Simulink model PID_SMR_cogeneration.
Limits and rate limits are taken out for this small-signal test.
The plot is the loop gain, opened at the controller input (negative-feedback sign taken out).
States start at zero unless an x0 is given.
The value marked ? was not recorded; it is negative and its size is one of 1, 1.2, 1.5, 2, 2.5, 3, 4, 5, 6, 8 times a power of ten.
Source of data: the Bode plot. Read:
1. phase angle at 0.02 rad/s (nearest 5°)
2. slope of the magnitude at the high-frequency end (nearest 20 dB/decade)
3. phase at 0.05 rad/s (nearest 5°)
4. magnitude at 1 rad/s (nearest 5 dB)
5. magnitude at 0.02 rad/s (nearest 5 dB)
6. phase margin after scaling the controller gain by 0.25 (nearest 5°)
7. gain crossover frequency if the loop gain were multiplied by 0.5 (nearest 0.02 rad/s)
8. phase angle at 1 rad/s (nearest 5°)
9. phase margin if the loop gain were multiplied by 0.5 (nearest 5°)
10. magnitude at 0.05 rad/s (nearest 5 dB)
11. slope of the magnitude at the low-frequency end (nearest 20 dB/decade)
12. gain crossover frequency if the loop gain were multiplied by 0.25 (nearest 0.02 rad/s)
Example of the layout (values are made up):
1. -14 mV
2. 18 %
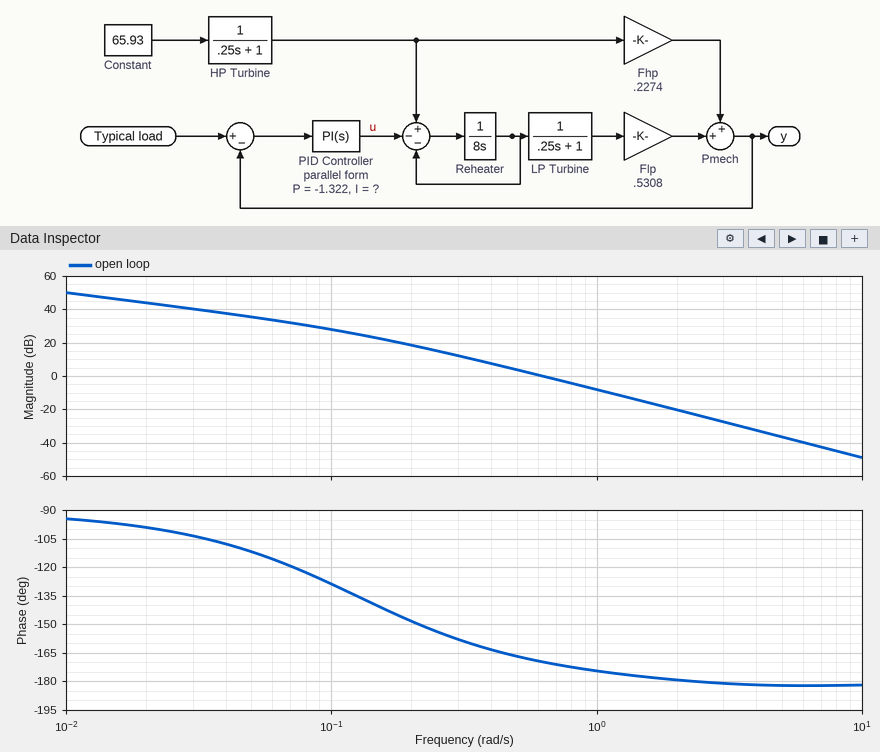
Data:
1. -100°
2. -40 dB/decade
3. -110°
4. -10 dB
5. 45 dB
6. 20°
7. 0.44 rad/s
8. -175°
9. 15°
10. 35 dB
11. -20 dB/decade
12. 0.30 rad/s
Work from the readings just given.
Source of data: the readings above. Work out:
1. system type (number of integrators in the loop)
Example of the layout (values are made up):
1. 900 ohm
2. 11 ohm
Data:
1. 1
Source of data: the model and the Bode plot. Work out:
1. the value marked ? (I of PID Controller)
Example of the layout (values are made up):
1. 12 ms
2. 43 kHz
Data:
1. -6
